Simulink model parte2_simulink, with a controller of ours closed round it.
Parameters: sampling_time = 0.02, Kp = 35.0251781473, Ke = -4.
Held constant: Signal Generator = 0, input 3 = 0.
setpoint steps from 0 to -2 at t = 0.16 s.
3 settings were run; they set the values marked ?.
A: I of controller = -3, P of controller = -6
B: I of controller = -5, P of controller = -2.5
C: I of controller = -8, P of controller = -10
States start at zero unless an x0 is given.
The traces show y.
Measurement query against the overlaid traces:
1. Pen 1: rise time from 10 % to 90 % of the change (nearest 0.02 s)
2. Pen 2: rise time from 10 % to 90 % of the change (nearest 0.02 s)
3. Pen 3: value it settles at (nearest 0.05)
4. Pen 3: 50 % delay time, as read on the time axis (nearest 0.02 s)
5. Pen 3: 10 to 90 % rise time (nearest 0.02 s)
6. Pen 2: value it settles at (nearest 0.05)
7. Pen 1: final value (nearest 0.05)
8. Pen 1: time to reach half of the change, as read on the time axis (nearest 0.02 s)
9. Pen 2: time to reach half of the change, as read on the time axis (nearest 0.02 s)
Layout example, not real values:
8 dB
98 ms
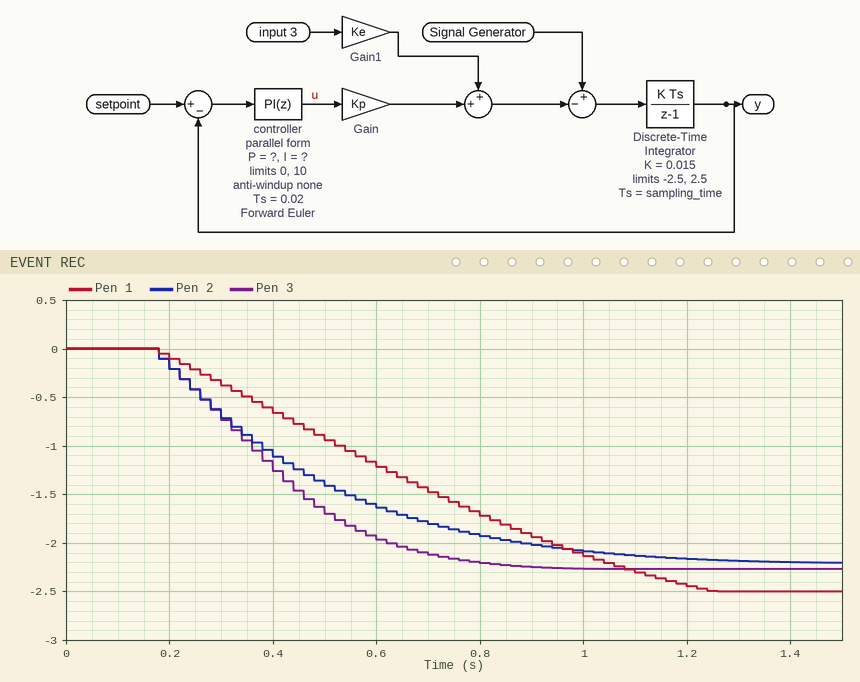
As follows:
0.82 s
0.64 s
-2.25
0.38 s
0.44 s
-2.20
-2.50
0.62 s
0.40 s
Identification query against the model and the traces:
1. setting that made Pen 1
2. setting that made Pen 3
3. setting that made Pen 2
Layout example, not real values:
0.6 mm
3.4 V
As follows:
B
C
A
